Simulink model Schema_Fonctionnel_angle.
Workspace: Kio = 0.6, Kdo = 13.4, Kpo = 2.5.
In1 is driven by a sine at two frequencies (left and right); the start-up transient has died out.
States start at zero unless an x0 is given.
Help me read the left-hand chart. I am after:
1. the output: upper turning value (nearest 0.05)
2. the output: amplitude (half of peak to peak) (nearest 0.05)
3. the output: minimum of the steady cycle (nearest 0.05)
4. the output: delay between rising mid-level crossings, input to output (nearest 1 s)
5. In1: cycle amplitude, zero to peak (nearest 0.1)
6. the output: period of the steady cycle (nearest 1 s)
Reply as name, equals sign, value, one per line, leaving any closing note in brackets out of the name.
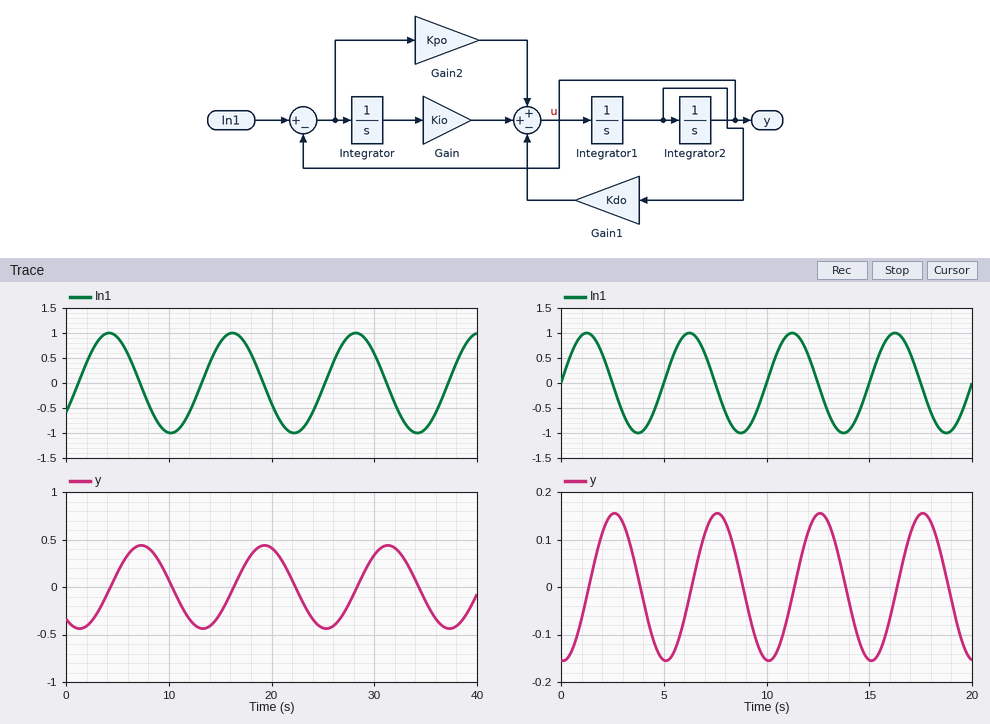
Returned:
the output: upper turning value = 0.45
the output: amplitude (half of peak to peak) = 0.45
the output: minimum of the steady cycle = -0.45
the output: delay between rising mid-level crossings, input to output = 3 s
In1: cycle amplitude, zero to peak = 1.0
the output: period of the steady cycle = 12 s
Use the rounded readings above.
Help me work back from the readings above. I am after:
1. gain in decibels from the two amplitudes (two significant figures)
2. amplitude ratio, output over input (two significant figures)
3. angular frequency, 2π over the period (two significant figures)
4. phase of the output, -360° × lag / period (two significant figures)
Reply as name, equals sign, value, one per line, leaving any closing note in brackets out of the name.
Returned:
gain in decibels from the two amplitudes = -6.9 dB
amplitude ratio, output over input = 0.45
angular frequency, 2π over the period = 0.52 rad/s
phase of the output, -360° × lag / period = -90°
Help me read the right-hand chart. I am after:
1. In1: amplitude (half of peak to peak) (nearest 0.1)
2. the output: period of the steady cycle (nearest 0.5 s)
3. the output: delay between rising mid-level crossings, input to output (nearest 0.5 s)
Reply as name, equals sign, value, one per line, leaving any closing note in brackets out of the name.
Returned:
In1: amplitude (half of peak to peak) = 1.0
the output: period of the steady cycle = 5.0 s
the output: delay between rising mid-level crossings, input to output = 1.5 s
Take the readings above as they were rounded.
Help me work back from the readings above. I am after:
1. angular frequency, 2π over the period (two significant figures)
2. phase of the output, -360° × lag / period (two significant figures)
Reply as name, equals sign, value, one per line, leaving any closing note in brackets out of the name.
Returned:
angular frequency, 2π over the period = 1.3 rad/s
phase of the output, -360° × lag / period = -110°
